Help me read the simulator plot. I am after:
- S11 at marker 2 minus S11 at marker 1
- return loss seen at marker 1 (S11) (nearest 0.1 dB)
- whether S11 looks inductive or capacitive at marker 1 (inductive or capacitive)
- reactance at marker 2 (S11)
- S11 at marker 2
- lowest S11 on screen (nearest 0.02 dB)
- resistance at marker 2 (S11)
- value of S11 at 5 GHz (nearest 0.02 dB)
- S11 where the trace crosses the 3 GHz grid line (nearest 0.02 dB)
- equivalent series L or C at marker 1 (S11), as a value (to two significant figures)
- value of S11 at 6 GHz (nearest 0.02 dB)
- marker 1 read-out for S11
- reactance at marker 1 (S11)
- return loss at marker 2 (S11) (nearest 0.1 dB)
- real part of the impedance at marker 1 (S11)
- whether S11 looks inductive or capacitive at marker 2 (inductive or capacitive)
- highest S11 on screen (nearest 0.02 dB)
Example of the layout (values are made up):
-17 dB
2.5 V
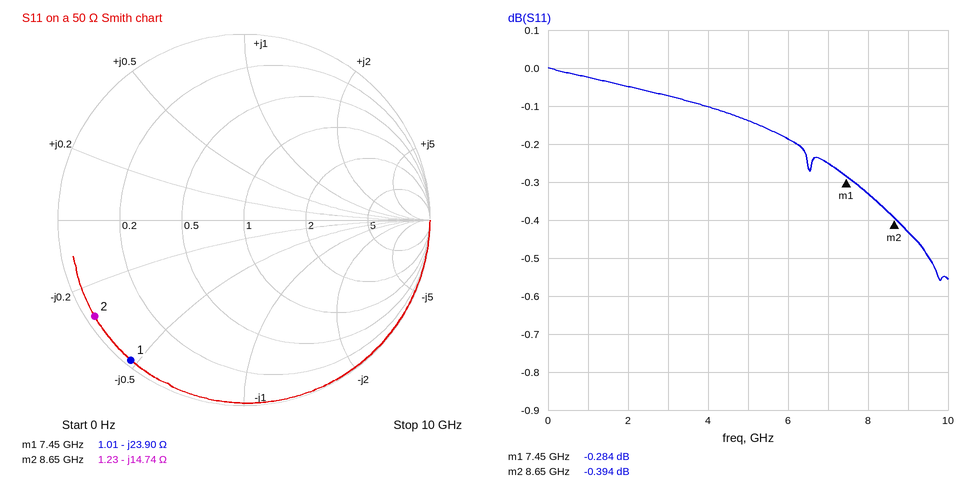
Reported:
-0.110 dB
0.3 dB
capacitive
-14.74 Ω
-0.394 dB
-0.56 dB
1.23 Ω
-0.14 dB
-0.08 dB
890 fF
-0.18 dB
-0.284 dB
-23.90 Ω
0.4 dB
1.01 Ω
capacitive
0.00 dB
